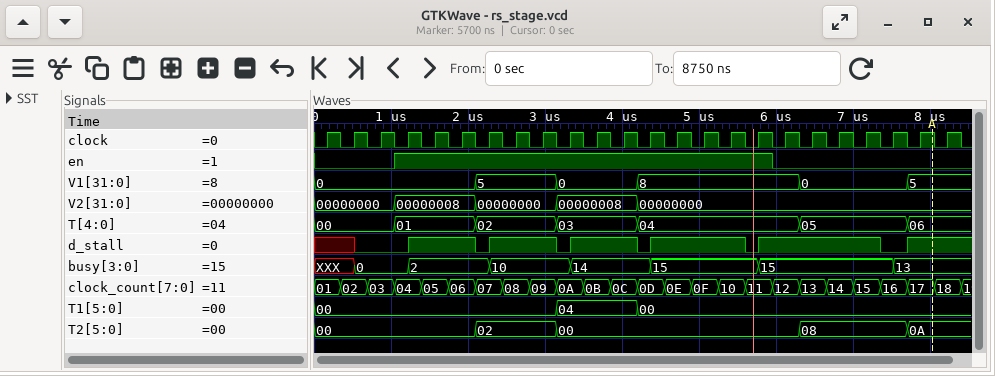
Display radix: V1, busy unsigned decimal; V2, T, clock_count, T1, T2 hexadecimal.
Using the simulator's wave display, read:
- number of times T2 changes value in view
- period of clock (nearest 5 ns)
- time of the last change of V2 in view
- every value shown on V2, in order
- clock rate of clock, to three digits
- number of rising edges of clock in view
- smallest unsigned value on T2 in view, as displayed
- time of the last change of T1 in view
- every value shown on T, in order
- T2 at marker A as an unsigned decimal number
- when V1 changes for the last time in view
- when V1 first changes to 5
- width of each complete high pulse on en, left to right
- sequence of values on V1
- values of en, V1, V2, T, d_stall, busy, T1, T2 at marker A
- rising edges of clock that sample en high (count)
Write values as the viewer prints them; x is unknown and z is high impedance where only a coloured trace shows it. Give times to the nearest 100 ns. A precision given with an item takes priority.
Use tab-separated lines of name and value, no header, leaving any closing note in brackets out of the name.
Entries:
number of times T2 changes value in view	4
period of clock	350 ns
time of the last change of V2 in view	4200 ns
every value shown on V2, in order	00000000, 00000008, 00000000, 00000008, 00000000
clock rate of clock, to three digits	2.86 MHz
number of rising edges of clock in view	24
smallest unsigned value on T2 in view, as displayed	00
time of the last change of T1 in view	4200 ns
every value shown on T, in order	00, 01, 02, 03, 04, 05, 06
T2 at marker A as an unsigned decimal number	10
when V1 changes for the last time in view	7700 ns
when V1 first changes to 5	2100 ns
width of each complete high pulse on en, left to right	4900 ns
sequence of values on V1	0, 5, 0, 8, 0, 5
values of en, V1, V2, T, d_stall, busy, T1, T2 at marker A	en=0, V1=5, V2=00000000, T=06, d_stall=1, busy=13, T1=00, T2=0A
rising edges of clock that sample en high	14
